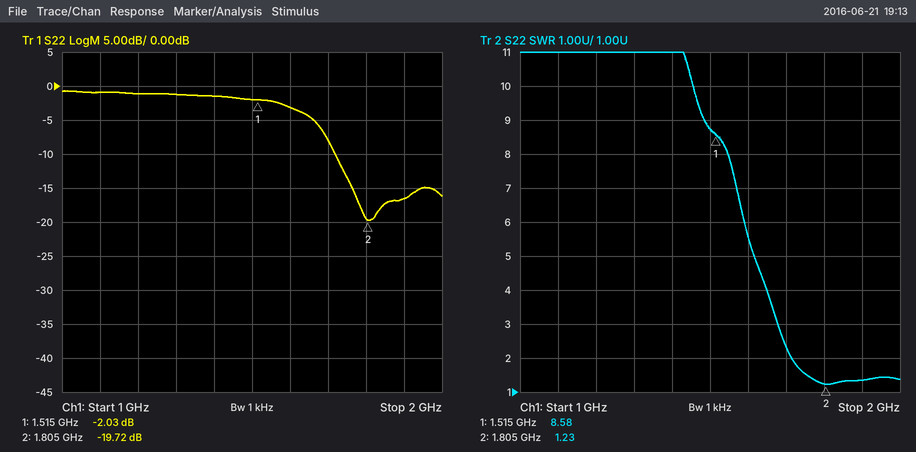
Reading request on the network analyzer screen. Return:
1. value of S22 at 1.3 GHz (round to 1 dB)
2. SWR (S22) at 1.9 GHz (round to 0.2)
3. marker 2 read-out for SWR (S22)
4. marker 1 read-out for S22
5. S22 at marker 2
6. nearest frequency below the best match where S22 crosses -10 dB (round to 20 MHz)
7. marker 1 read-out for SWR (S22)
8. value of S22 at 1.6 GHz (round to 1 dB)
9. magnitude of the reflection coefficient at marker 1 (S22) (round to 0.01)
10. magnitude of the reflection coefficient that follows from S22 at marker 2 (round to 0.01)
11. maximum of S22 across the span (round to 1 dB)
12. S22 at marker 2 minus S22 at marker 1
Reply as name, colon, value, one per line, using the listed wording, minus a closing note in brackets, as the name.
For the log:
value of S22 at 1.3 GHz: -1 dB
SWR (S22) at 1.9 GHz: 1.4
marker 2 read-out for SWR: 1.23
marker 1 read-out for S22: -2.03 dB
S22 at marker 2: -19.72 dB
nearest frequency below the best match where S22 crosses -10 dB: 1.72 GHz
marker 1 read-out for SWR: 8.58
value of S22 at 1.6 GHz: -3 dB
magnitude of the reflection coefficient at marker 1 (S22): 0.79
magnitude of the reflection coefficient that follows from S22 at marker 2: 0.10
maximum of S22 across the span: -1 dB
S22 at marker 2 minus S22 at marker 1: -17.69 dB
